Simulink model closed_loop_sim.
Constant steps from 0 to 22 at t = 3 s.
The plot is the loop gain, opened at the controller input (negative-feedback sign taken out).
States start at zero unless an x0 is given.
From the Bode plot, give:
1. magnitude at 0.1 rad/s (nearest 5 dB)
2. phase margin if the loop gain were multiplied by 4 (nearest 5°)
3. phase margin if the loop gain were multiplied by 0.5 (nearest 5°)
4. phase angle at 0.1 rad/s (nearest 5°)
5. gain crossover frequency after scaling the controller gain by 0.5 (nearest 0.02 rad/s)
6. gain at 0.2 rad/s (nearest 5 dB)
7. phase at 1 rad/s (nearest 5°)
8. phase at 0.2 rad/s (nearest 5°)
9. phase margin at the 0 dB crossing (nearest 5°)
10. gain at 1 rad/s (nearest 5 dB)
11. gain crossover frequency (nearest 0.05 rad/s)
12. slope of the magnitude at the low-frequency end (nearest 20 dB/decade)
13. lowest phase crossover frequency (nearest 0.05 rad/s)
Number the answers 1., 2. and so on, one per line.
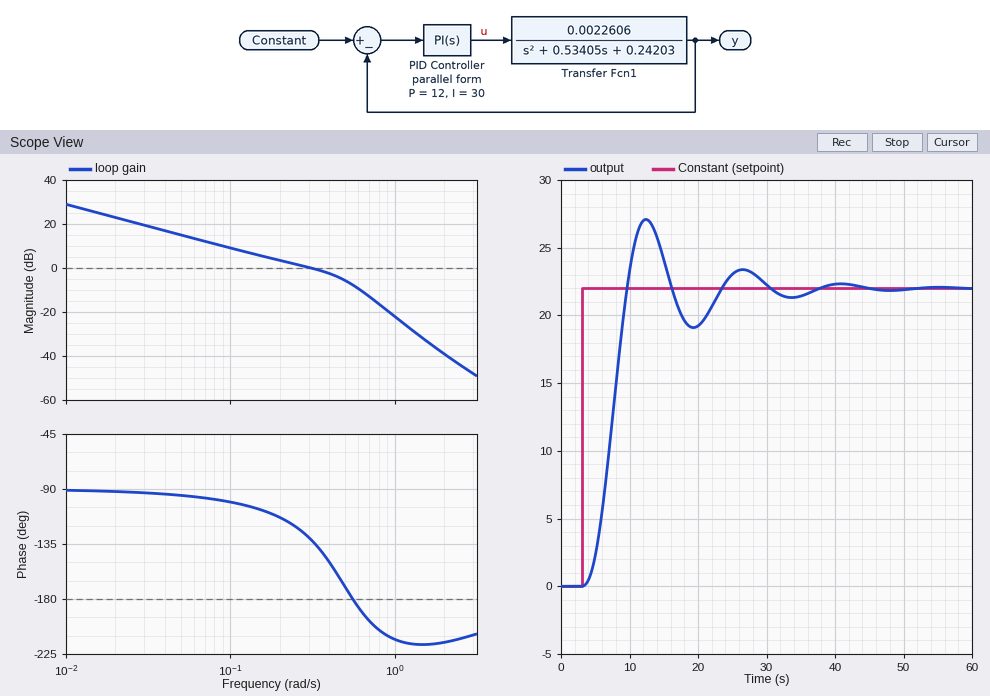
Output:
1. 10 dB
2. -15°
3. 75°
4. -100°
5. 0.14 rad/s
6. 5 dB
7. -215°
8. -115°
9. 50°
10. -20 dB
11. 0.30 rad/s
12. -20 dB/decade
13. 0.55 rad/s
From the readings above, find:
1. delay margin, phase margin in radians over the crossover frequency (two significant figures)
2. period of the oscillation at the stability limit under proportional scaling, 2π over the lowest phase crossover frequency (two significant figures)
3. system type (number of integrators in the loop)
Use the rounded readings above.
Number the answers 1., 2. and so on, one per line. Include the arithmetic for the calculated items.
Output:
1. 50 × π / 180 / 0.3 = 2.9 s
2. 2π / 0.55 = 11 s
3. 1
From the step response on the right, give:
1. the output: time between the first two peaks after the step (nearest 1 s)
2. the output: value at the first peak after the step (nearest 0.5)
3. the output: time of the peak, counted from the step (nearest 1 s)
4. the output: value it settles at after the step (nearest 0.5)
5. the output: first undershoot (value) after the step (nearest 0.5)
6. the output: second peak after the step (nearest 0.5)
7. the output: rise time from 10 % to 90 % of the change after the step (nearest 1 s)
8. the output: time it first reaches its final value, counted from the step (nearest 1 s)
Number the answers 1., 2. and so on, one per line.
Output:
1. 14 s
2. 27.0
3. 9 s
4. 22.0
5. 19.0
6. 23.5
7. 4 s
8. 7 s
